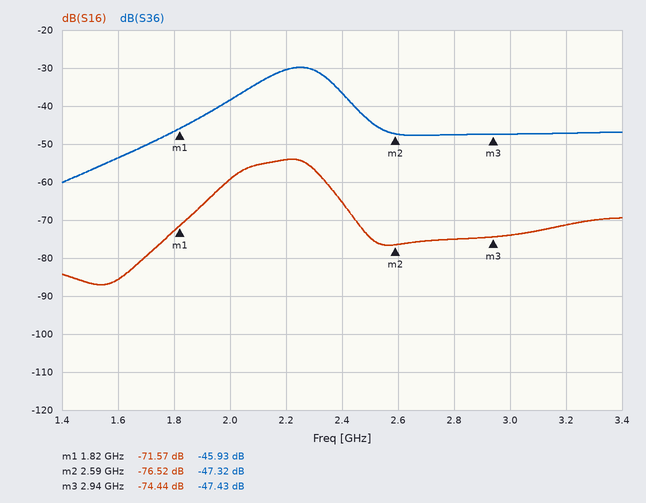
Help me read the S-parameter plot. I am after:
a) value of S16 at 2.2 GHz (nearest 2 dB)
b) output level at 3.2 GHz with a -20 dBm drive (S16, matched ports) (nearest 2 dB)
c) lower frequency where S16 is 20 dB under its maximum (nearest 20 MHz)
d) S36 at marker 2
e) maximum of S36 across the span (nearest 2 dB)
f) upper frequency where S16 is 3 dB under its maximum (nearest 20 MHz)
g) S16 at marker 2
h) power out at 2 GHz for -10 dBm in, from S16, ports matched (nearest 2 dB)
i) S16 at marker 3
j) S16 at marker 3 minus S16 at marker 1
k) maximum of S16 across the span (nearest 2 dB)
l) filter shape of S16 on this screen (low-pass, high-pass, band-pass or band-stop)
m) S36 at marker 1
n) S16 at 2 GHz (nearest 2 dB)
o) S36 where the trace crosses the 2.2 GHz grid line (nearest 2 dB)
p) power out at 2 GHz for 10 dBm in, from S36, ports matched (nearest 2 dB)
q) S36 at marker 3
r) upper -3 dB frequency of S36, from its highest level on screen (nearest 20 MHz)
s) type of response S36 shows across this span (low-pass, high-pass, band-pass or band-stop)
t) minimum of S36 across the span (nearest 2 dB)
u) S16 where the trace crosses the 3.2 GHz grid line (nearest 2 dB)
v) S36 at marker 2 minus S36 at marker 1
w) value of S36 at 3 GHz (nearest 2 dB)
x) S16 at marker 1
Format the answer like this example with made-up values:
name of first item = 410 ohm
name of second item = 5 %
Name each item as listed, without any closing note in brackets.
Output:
value of S16 at 2.2 GHz = -54 dB
output level at 3.2 GHz with a -20 dBm drive (S16, matched ports) = -92 dBm
lower frequency where S16 is 20 dB under its maximum = 1.78 GHz
S36 at marker 2 = -47.32 dB
maximum of S36 across the span = -30 dB
upper frequency where S16 is 3 dB under its maximum = 2.30 GHz
S16 at marker 2 = -76.52 dB
power out at 2 GHz for -10 dBm in, from S16, ports matched = -70 dBm
S16 at marker 3 = -74.44 dB
S16 at marker 3 minus S16 at marker 1 = -2.87 dB
maximum of S16 across the span = -54 dB
filter shape of S16 on this screen = band-pass
S36 at marker 1 = -45.93 dB
S16 at 2 GHz = -60 dB
S36 where the trace crosses the 2.2 GHz grid line = -30 dB
power out at 2 GHz for 10 dBm in, from S36, ports matched = -28 dBm
S36 at marker 3 = -47.43 dB
upper -3 dB frequency of S36, from its highest level on screen = 2.34 GHz
type of response S36 shows across this span = band-pass
minimum of S36 across the span = -60 dB
S16 where the trace crosses the 3.2 GHz grid line = -72 dB
S36 at marker 2 minus S36 at marker 1 = -1.39 dB
value of S36 at 3 GHz = -48 dB
S16 at marker 1 = -71.57 dB
